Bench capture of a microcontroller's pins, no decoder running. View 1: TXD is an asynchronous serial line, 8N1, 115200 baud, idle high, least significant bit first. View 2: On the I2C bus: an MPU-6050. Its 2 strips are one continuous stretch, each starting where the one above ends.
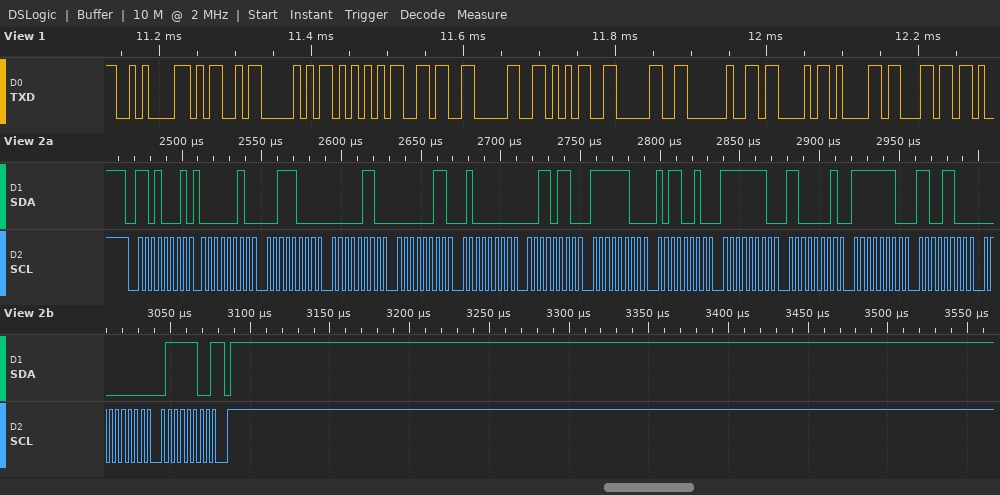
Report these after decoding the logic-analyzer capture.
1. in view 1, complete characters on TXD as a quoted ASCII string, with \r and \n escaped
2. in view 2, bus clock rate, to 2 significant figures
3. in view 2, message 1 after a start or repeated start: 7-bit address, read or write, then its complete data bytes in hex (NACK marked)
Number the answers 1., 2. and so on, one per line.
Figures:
1. "\nMPU6050 Cal"
2. 250 kHz
3. 0x68 read: 02 38 06 03 40 36 FC B2 FE C1 FE CC 00 7C NACK
